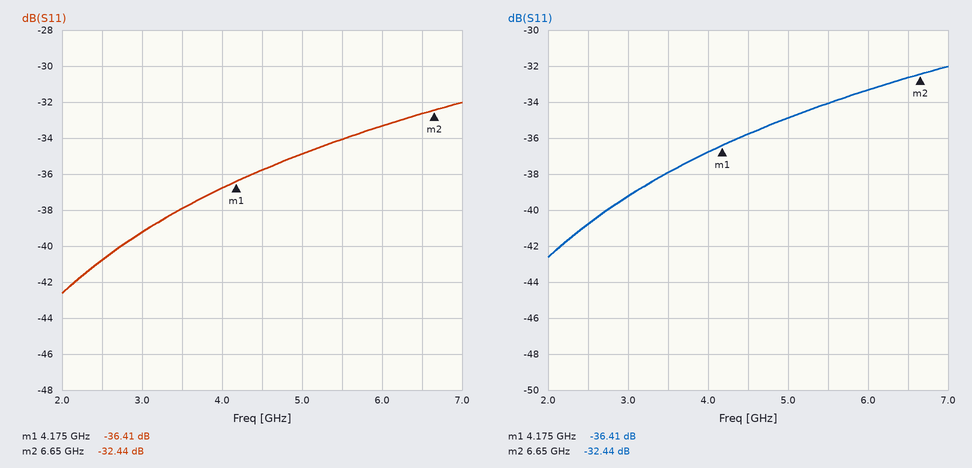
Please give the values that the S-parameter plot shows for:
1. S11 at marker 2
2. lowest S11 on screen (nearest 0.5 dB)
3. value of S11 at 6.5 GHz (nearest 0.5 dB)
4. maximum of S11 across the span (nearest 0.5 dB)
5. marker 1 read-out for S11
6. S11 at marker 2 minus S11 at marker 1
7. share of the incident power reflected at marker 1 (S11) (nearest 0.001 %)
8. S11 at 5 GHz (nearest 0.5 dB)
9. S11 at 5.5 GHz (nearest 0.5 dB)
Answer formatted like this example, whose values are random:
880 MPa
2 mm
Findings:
-32.44 dB
-42.5 dB
-32.5 dB
-32.0 dB
-36.41 dB
3.97 dB
0.023 %
-35.0 dB
-34.0 dB
